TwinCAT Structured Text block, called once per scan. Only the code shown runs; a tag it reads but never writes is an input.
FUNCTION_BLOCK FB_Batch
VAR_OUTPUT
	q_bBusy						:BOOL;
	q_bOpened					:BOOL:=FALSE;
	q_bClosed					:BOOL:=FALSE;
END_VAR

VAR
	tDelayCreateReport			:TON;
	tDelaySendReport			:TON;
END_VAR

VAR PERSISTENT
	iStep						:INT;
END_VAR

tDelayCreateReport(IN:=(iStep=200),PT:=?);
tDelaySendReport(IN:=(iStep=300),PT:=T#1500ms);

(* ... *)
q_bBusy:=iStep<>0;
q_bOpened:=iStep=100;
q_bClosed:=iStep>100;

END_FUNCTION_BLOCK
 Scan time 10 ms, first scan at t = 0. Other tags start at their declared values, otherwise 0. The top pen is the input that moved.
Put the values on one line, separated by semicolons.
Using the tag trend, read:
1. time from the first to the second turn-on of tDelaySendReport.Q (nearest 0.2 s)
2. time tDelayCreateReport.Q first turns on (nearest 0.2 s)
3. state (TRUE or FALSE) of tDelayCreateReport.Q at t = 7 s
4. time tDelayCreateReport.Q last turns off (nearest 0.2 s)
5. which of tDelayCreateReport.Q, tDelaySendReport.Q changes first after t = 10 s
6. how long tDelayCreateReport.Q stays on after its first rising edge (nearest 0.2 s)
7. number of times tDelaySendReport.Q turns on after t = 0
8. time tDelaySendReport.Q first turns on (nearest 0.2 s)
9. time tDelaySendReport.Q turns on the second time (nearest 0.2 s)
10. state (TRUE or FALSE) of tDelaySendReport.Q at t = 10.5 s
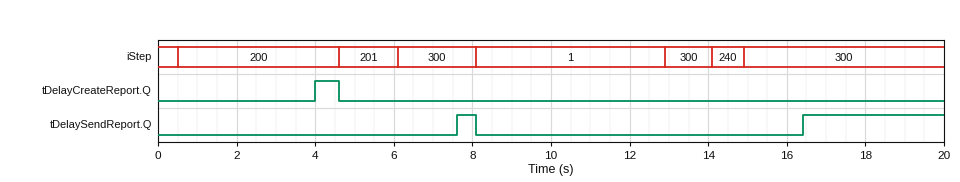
8.8 s; 4.0 s; FALSE; 4.6 s; tDelaySendReport.Q; 0.6 s; 2; 7.6 s; 16.4 s; FALSE
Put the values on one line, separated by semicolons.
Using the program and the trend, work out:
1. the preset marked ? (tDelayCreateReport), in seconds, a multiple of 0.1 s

3.5 s
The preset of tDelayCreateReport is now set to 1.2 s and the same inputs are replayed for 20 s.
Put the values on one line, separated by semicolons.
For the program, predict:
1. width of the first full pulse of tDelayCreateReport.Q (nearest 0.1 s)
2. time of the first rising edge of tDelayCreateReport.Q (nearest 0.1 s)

2.9 s; 1.7 s
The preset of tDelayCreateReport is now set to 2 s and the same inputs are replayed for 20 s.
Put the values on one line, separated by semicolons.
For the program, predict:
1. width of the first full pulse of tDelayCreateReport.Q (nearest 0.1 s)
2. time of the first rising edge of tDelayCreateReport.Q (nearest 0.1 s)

2.1 s; 2.5 s
